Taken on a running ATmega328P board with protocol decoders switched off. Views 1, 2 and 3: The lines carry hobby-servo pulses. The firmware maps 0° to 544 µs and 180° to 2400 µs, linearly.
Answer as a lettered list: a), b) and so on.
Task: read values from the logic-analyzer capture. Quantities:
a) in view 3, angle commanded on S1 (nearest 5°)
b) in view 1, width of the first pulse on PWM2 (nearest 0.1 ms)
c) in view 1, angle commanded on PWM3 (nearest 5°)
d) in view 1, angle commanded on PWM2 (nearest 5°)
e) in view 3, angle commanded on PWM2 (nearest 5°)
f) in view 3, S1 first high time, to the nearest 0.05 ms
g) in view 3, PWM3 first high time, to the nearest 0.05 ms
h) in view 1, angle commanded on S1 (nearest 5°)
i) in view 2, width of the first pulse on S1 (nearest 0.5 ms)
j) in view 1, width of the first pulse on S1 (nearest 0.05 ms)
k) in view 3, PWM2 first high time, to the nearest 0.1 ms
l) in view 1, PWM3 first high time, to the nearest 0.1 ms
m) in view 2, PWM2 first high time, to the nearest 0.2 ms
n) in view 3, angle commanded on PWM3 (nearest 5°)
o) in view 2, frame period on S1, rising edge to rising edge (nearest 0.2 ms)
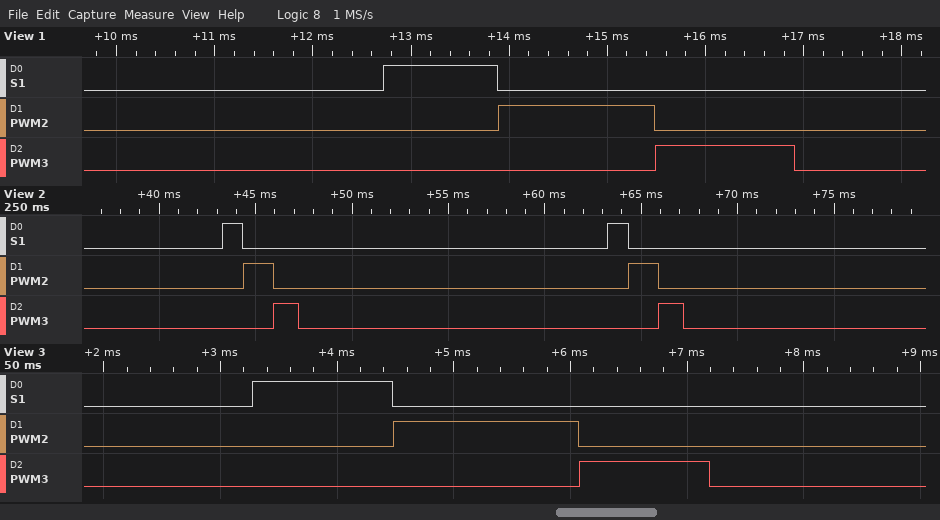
a) 65°
b) 1.6 ms
c) 85°
d) 100°
e) 100°
f) 1.20 ms
g) 1.10 ms
h) 60°
i) 1.0 ms
j) 1.15 ms
k) 1.6 ms
l) 1.4 ms
m) 1.6 ms
n) 55°
o) 20.0 ms
